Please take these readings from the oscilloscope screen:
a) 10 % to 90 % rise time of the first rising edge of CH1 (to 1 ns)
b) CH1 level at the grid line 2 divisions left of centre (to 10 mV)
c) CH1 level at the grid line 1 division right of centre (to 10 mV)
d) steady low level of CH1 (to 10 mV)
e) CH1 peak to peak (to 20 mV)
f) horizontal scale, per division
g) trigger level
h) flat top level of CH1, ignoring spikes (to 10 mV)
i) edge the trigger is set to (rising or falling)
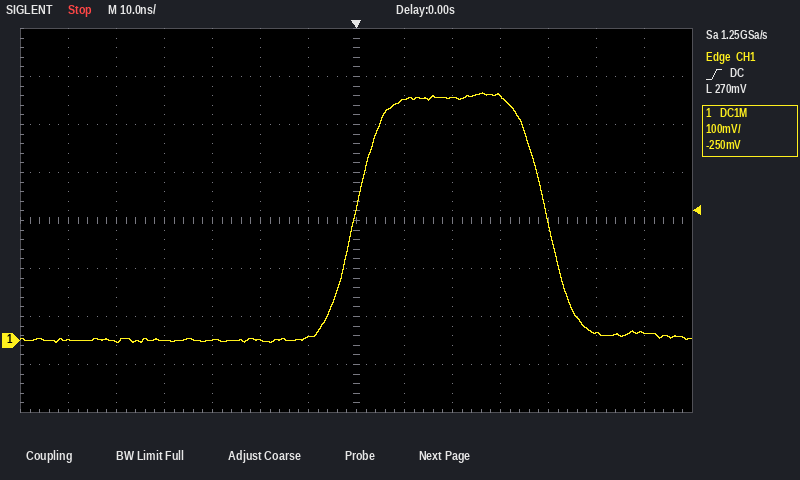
11 ns
0 mV
500 mV
0 mV
520 mV
10 ns
270 mV
510 mV
rising
